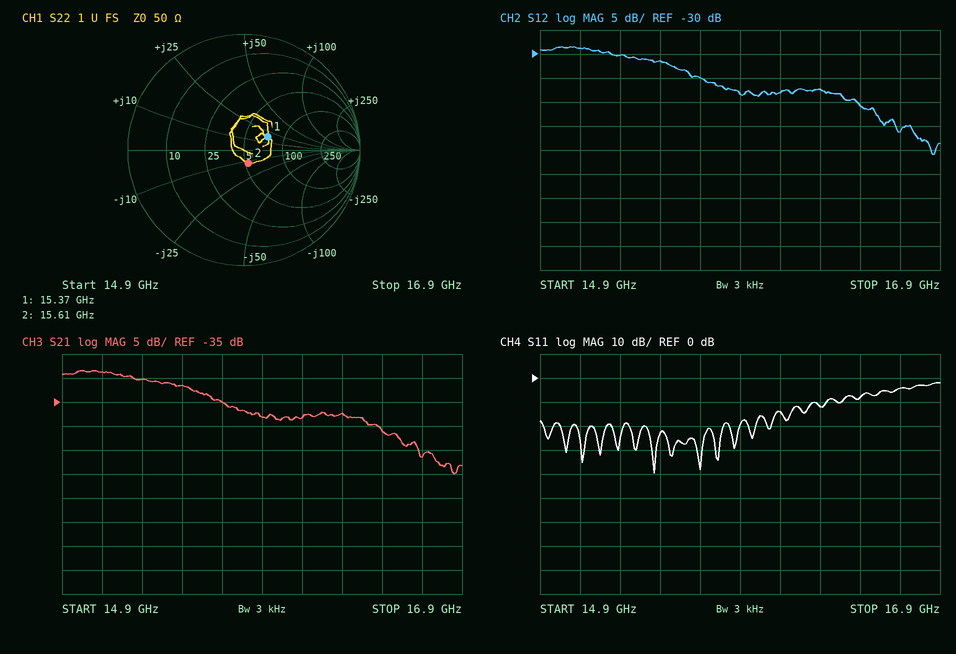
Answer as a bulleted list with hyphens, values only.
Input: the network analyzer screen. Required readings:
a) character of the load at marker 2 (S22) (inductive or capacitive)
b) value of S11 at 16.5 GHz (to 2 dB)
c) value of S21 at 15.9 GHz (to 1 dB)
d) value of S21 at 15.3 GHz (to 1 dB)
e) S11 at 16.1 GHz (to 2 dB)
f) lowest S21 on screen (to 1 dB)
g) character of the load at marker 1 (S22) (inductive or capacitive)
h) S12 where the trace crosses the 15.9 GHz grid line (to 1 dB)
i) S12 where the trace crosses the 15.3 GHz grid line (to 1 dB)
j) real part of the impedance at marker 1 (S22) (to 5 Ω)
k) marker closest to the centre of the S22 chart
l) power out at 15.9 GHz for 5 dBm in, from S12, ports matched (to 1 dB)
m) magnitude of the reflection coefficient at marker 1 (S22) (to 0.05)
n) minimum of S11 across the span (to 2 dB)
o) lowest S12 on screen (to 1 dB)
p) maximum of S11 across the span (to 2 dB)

- capacitive
- -8 dB
- -38 dB
- -30 dB
- -14 dB
- -50 dB
- inductive
- -38 dB
- -30 dB
- 75 Ω
- marker 2
- -33 dBm
- 0.25
- -40 dB
- -51 dB
- -2 dB
